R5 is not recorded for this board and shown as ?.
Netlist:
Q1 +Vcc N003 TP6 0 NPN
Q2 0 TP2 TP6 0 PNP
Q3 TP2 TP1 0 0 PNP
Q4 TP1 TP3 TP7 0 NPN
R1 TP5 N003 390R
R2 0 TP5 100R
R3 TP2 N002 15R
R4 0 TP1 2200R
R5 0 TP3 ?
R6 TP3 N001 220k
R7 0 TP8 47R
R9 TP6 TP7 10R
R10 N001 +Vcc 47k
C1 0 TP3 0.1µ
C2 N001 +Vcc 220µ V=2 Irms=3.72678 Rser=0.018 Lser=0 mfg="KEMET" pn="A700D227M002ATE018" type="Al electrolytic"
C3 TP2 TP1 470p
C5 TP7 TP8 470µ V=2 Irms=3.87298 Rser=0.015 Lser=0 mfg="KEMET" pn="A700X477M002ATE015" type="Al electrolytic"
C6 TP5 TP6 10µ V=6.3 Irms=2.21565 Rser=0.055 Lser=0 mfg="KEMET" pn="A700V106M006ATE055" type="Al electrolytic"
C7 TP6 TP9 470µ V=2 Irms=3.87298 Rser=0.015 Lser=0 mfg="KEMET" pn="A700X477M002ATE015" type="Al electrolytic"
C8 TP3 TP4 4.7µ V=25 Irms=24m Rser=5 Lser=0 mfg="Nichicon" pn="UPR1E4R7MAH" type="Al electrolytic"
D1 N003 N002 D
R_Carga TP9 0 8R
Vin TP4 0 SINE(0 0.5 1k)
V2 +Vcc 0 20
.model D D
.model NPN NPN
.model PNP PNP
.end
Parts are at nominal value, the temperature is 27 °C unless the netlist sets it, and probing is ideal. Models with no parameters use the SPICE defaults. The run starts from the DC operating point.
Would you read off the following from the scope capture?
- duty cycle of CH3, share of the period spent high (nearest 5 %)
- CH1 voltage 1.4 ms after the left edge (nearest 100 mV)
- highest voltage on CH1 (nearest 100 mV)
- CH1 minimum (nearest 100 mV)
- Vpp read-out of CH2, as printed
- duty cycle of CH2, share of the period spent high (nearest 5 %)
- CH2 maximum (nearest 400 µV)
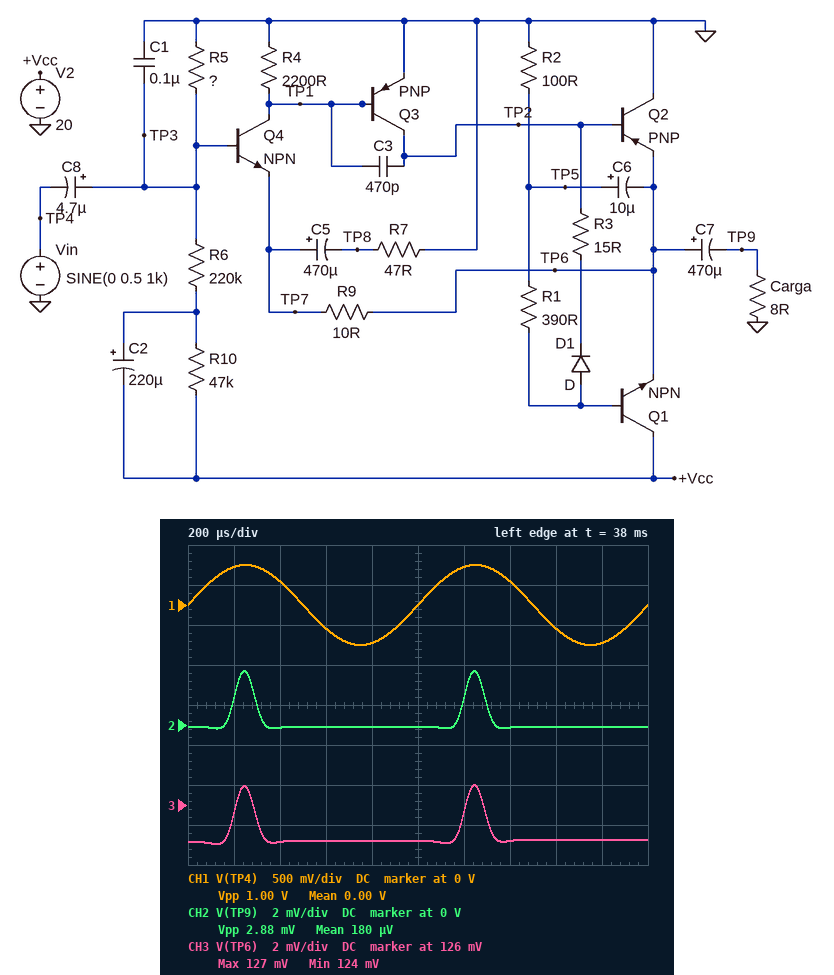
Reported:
10 %
300 mV
500 mV
-500 mV
2.88 mV
10 %
2.8 mV
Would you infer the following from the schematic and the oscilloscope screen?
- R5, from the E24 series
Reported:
47 kΩ
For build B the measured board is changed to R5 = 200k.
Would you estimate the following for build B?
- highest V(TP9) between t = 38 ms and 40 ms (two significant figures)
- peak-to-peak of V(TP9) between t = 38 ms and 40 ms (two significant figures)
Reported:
2.9 mV
3.1 mV
